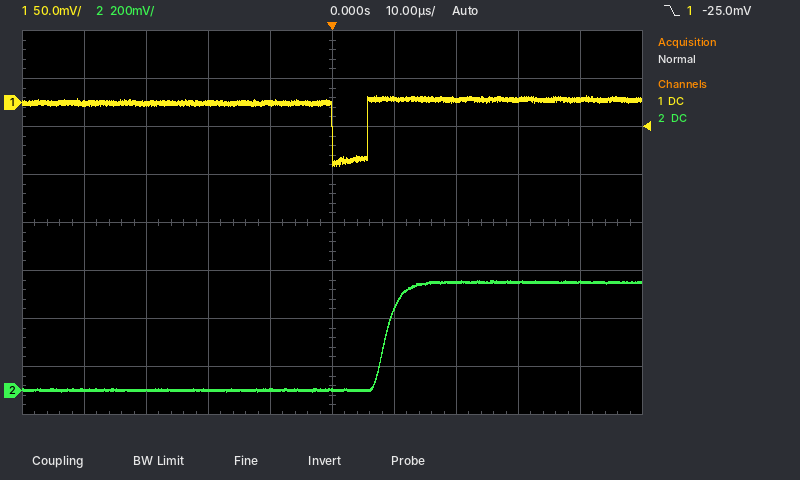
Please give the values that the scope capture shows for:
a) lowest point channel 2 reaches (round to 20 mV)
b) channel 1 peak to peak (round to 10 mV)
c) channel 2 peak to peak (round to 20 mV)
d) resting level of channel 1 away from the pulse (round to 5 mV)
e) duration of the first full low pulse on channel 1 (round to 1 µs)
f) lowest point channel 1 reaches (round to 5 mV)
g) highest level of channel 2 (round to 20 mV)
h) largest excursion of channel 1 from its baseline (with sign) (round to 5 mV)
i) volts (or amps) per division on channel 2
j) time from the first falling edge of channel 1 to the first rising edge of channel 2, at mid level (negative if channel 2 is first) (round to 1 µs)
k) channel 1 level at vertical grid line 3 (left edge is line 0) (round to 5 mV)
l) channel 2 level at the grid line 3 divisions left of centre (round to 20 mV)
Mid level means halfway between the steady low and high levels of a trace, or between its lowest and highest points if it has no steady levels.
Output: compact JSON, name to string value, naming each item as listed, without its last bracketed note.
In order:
{"lowest point channel 2 reaches": "0 mV", "channel 1 peak to peak": "70 mV", "channel 2 peak to peak": "460 mV", "resting level of channel 1 away from the pulse": "0 mV", "duration of the first full low pulse on channel 1": "6 µs", "lowest point channel 1 reaches": "-65 mV", "highest level of channel 2": "460 mV", "largest excursion of channel 1 from its baseline (with sign)": "-65 mV", "volts (or amps) per division on channel 2": "200 mV", "time from the first falling edge of channel 1 to the first rising edge of channel 2, at mid level (negative if channel 2 is first)": "+9 µs", "channel 1 level at vertical grid line 3 (left edge is line 0)": "0 mV", "channel 2 level at the grid line 3 divisions left of centre": "0 mV"}
